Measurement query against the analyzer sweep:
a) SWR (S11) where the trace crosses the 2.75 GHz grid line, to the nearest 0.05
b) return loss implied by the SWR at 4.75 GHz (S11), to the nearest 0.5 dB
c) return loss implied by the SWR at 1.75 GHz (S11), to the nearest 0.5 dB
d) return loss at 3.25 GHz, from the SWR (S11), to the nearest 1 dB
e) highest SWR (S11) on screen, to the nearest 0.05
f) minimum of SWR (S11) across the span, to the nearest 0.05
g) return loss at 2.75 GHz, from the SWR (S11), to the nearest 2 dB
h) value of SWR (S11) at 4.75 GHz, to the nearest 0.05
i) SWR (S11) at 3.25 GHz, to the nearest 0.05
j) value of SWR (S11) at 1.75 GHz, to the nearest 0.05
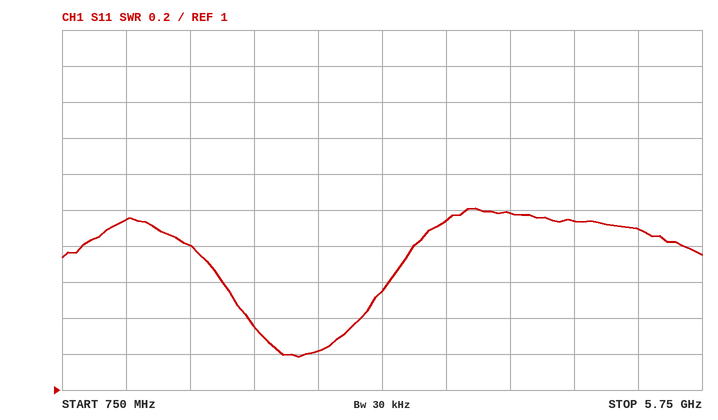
1.20
10.0 dB
11.0 dB
13 dB
2.00
1.20
20 dB
1.95
1.55
1.80
